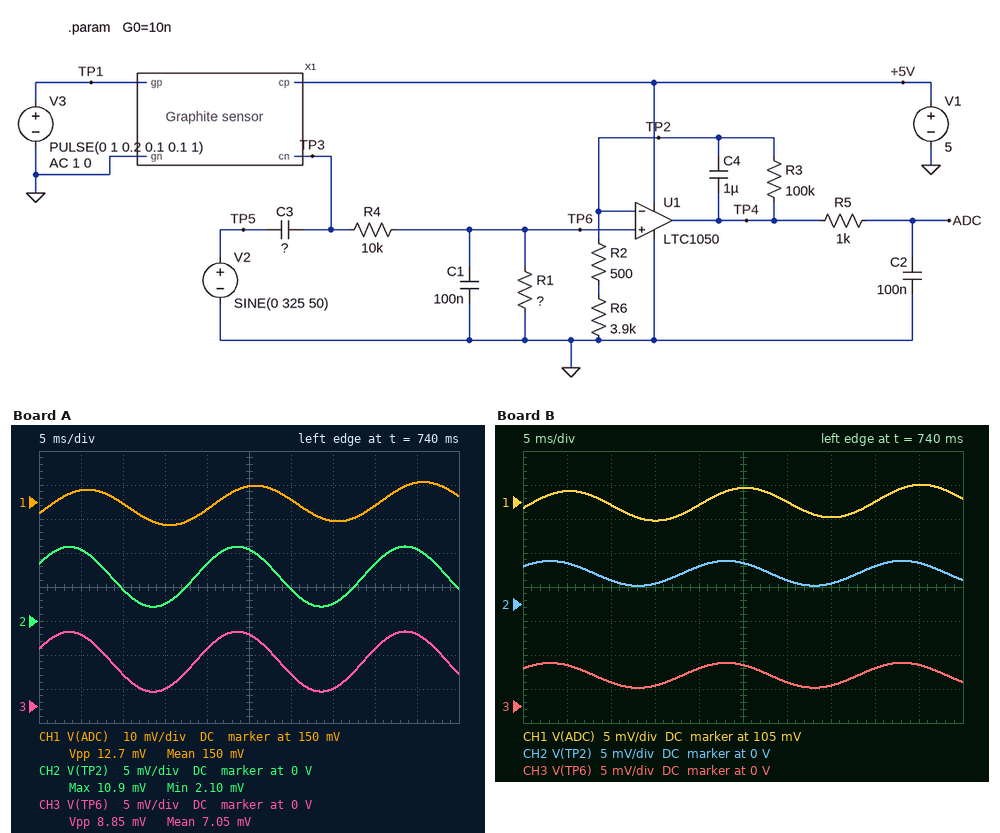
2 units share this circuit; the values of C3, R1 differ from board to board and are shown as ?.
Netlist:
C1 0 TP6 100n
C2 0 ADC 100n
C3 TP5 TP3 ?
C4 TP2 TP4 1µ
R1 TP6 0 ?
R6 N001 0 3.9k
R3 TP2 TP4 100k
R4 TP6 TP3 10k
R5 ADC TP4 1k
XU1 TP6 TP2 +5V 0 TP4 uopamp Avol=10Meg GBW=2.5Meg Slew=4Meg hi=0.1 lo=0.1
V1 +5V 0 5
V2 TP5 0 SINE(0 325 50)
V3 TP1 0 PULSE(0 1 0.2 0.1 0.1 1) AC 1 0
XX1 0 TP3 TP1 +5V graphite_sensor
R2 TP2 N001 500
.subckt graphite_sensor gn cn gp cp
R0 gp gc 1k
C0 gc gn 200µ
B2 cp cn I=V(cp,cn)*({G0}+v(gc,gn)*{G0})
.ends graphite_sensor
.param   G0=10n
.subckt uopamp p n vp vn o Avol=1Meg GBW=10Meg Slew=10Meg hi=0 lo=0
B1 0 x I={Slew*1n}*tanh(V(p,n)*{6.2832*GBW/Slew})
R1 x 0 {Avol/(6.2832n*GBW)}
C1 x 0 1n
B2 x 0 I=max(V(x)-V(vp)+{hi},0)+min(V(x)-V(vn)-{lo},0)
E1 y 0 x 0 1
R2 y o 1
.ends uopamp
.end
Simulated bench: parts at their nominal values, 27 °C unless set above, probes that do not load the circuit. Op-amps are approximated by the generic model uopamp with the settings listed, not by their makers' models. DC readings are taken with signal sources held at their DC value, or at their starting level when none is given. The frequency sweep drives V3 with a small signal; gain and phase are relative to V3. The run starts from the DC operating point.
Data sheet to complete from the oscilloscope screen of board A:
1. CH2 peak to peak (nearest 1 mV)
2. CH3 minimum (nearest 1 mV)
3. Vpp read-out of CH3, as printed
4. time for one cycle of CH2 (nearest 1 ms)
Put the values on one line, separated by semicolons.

9 mV; 2 mV; 8.85 mV; 20 ms
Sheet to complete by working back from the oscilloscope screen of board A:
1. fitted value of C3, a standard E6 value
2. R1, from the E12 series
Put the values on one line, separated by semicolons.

1.5 pF; 68 kΩ
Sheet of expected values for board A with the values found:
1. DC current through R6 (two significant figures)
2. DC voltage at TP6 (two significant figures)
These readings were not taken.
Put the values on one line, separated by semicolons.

960 nA; 3.4 mV
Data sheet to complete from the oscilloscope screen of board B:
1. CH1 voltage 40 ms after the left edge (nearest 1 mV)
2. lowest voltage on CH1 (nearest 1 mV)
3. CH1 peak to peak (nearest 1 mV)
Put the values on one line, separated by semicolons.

105 mV; 102 mV; 5 mV
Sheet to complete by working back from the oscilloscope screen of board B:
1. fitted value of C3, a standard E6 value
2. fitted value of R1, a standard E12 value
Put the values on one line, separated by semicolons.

680 fF; 47 kΩ
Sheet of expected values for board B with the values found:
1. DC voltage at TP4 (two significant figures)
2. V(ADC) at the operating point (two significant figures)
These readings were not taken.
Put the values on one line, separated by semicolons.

100 mV; 100 mV
